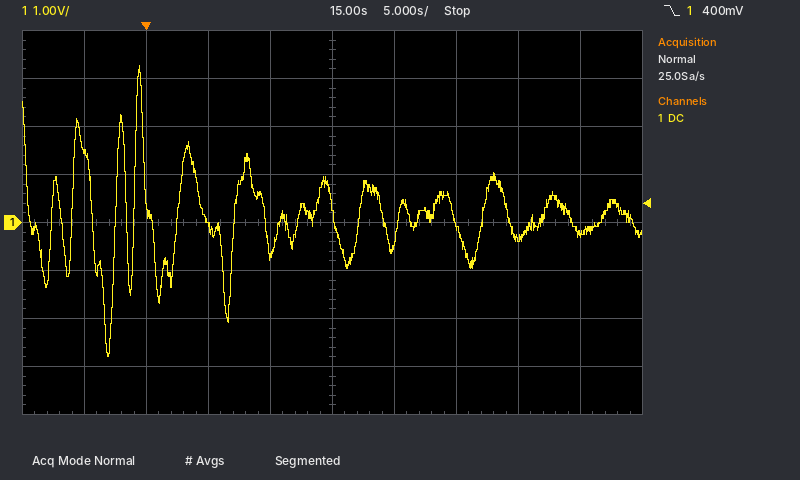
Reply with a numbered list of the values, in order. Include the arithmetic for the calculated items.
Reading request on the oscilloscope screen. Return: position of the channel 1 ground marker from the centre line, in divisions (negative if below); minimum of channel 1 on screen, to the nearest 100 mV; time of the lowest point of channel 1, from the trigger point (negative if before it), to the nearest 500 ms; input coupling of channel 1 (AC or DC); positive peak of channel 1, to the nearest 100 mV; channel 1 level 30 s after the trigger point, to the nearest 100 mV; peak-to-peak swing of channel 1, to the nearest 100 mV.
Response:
1. 0.0 div
2. -2.8 V
3. -3.0 s
4. DC
5. 3.3 V
6. -300 mV
7. 3.3 V − (-2.8 V) = 6.1 V
